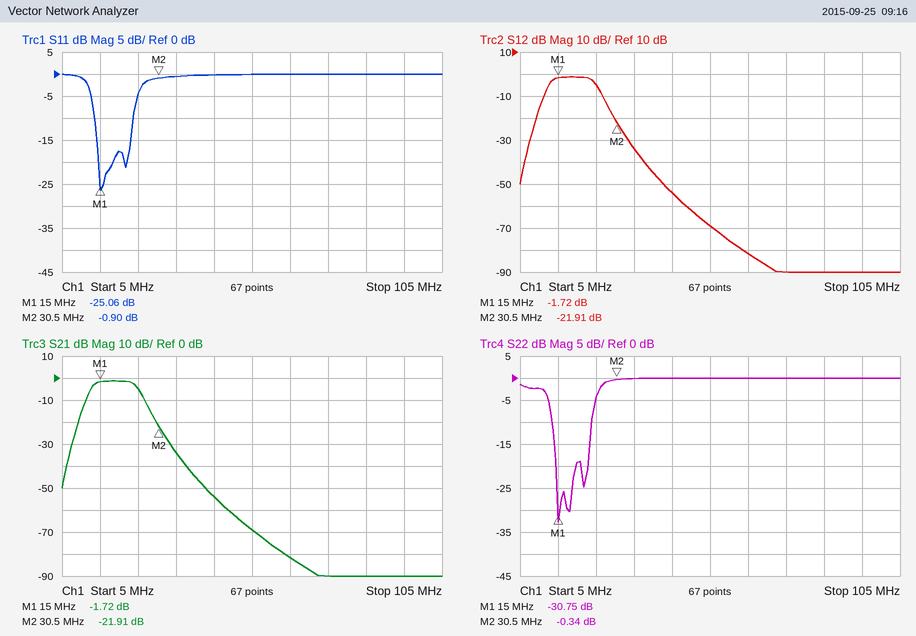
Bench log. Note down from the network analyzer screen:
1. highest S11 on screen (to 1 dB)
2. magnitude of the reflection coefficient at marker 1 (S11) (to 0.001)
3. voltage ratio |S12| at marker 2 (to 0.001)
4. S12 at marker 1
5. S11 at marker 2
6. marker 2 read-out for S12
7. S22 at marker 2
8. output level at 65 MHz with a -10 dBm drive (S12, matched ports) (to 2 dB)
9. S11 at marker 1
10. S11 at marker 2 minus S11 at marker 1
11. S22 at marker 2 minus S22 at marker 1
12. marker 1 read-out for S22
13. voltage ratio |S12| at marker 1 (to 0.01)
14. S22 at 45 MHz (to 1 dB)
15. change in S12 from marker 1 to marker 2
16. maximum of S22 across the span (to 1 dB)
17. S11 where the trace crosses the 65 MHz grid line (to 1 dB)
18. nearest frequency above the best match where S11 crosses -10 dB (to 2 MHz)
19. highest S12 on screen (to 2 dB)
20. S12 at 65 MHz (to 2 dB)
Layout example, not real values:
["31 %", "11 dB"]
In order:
["0 dB", "0.056", "0.080", "-1.72 dB", "-0.90 dB", "-21.91 dB", "-0.34 dB", "-92 dBm", "-25.06 dB", "24.16 dB", "30.41 dB", "-30.75 dB", "0.82", "0 dB", "-20.19 dB", "0 dB", "0 dB", "24 MHz", "-2 dB", "-82 dB"]
